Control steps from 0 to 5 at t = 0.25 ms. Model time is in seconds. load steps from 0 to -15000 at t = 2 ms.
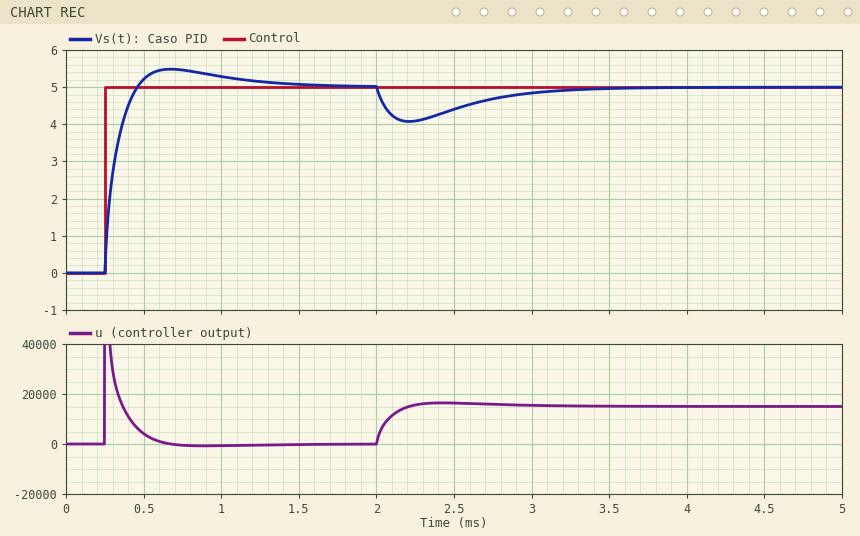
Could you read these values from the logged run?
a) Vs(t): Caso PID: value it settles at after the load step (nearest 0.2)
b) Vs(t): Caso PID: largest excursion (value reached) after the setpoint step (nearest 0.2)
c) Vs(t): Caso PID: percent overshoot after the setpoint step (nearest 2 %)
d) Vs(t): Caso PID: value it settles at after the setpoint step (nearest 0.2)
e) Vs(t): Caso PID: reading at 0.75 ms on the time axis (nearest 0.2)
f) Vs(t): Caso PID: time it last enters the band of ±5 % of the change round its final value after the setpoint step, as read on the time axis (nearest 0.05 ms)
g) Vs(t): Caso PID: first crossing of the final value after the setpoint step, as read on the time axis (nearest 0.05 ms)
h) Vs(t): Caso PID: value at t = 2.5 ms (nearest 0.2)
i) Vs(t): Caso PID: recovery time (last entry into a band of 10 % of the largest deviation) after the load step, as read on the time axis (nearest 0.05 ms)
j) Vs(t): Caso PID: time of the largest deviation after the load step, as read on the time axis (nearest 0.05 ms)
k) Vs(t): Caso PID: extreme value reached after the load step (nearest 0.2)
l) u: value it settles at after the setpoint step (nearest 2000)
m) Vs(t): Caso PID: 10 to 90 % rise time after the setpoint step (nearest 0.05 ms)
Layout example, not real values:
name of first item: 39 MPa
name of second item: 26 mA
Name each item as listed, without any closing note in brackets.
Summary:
Vs(t): Caso PID: value it settles at after the load step: 5.0
Vs(t): Caso PID: largest excursion (value reached) after the setpoint step: 5.4
Vs(t): Caso PID: percent overshoot after the setpoint step: 10 %
Vs(t): Caso PID: value it settles at after the setpoint step: 5.0
Vs(t): Caso PID: reading at 0.75 ms on the time axis: 5.4
Vs(t): Caso PID: time it last enters the band of ±5 % of the change round its final value after the setpoint step, as read on the time axis: 1.05 ms
Vs(t): Caso PID: first crossing of the final value after the setpoint step, as read on the time axis: 0.45 ms
Vs(t): Caso PID: value at t = 2.5 ms: 4.4
Vs(t): Caso PID: recovery time (last entry into a band of 10 % of the largest deviation) after the load step, as read on the time axis: 3.20 ms
Vs(t): Caso PID: time of the largest deviation after the load step, as read on the time axis: 2.20 ms
Vs(t): Caso PID: extreme value reached after the load step: 4.0
u: value it settles at after the setpoint step: 0
Vs(t): Caso PID: 10 to 90 % rise time after the setpoint step: 0.15 ms
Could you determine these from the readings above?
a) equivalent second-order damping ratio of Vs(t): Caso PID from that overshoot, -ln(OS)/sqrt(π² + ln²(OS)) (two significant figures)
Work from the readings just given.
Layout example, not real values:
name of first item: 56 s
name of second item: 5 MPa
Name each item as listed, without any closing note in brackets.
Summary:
equivalent second-order damping ratio of Vs(t): Caso PID from that overshoot, -ln(OS)/sqrt(π² + ln²(OS)): 0.59
